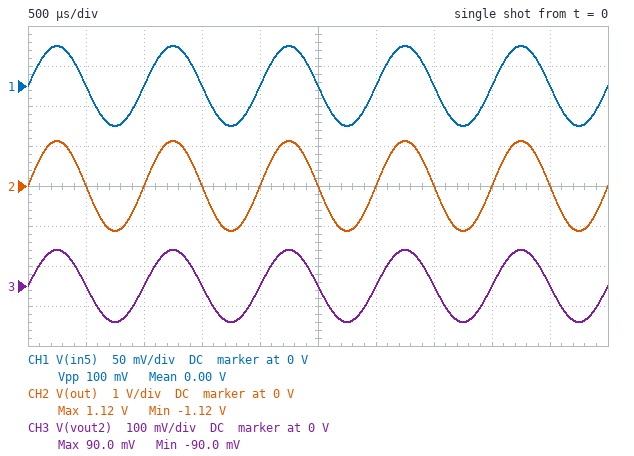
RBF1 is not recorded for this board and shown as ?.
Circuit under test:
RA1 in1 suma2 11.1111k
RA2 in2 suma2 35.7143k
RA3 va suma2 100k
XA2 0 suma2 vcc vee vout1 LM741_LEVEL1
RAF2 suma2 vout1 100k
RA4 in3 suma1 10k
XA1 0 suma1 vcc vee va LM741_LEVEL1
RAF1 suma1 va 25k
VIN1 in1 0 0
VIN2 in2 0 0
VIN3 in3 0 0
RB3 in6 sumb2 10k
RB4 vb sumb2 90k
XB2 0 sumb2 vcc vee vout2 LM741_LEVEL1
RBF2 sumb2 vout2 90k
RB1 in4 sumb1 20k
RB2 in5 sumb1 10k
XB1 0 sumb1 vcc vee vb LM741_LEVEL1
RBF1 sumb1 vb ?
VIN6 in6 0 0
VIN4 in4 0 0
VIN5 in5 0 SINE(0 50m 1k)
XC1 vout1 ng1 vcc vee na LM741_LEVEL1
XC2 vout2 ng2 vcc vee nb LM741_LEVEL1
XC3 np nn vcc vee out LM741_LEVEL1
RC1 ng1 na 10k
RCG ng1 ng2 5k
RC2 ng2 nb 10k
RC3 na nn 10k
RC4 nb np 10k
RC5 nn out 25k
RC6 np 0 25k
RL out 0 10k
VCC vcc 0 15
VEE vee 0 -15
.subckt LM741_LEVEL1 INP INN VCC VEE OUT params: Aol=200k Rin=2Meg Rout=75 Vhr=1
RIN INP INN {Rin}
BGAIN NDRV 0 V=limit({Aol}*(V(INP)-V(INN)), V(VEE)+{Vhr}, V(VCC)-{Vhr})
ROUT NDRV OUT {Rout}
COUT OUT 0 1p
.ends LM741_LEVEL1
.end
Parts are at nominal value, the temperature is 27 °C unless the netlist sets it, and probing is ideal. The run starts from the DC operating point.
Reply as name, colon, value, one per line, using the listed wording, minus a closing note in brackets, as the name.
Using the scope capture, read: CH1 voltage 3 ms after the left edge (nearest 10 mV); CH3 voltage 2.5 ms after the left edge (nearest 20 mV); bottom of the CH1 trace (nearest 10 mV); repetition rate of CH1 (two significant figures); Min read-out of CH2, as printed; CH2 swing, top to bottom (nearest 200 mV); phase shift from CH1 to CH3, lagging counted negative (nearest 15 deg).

CH1 voltage 3 ms after the left edge: 0 V
CH3 voltage 2.5 ms after the left edge: 0 V
bottom of the CH1 trace: -50 mV
repetition rate of CH1: 1.0 kHz
Min read-out of CH2, as printed: -1.12 V
CH2 swing, top to bottom: 2.2 V
phase shift from CH1 to CH3, lagging counted negative: 0 deg
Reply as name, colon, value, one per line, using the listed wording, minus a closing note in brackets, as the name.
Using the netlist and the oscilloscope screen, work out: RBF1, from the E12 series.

RBF1, from the E12 series: 18 kΩ
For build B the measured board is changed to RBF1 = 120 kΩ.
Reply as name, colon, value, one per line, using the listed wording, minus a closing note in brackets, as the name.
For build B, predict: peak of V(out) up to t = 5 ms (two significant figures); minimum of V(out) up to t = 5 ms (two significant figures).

peak of V(out) up to t = 5 ms: 7.5 V
minimum of V(out) up to t = 5 ms: -7.5 V
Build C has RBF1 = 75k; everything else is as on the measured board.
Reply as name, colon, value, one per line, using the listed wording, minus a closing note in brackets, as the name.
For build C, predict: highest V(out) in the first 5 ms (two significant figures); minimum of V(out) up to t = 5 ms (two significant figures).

highest V(out) in the first 5 ms: 4.7 V
minimum of V(out) up to t = 5 ms: -4.7 V
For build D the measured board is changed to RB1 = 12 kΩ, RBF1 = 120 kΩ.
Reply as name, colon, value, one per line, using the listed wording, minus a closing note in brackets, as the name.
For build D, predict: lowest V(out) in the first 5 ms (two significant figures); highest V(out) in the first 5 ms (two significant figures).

lowest V(out) in the first 5 ms: -7.5 V
highest V(out) in the first 5 ms: 7.5 V
